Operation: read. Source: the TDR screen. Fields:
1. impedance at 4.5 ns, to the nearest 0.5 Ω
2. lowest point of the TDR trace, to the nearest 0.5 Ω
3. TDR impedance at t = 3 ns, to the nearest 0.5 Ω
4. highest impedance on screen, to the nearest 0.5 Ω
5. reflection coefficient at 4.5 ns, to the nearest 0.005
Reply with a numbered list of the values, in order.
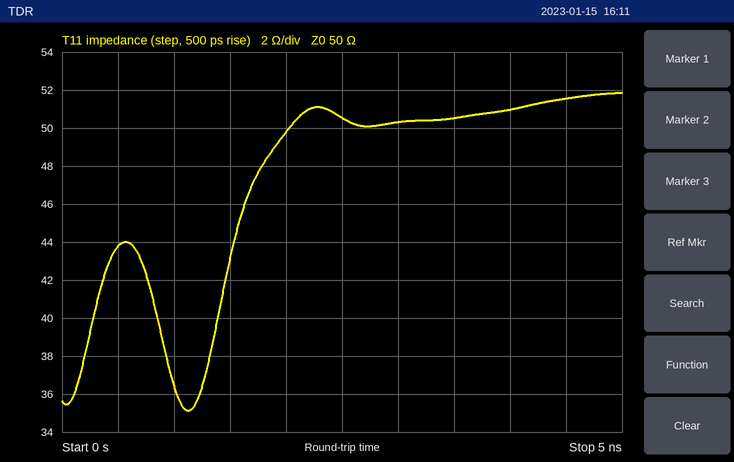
1. 51.5 Ω
2. 35.0 Ω
3. 50.5 Ω
4. 52.0 Ω
5. +0.015
